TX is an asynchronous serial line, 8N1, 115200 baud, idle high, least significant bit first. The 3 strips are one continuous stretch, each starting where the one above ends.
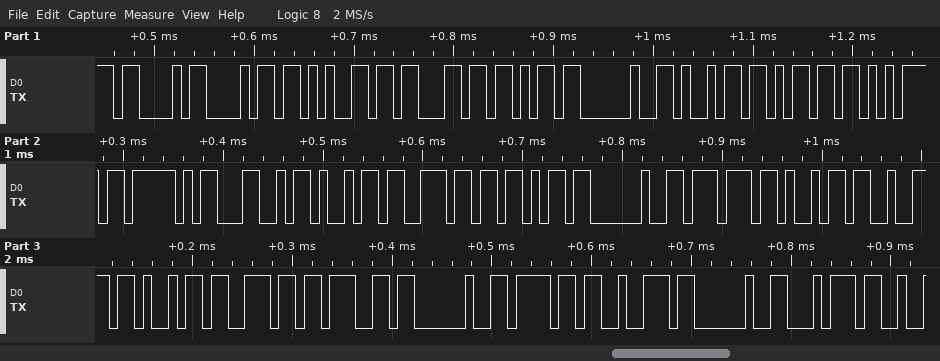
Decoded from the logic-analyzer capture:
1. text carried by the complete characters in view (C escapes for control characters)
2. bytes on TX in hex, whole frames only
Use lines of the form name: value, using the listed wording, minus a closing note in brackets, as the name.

text carried by the complete characters in view: "Check imu_Link wiring or t"
bytes on TX in hex, whole frames only: 43 68 65 63 6B 20 69 6D 75 5F 4C 69 6E 6B 20 77 69 72 69 6E 67 20 6F 72 20 74
